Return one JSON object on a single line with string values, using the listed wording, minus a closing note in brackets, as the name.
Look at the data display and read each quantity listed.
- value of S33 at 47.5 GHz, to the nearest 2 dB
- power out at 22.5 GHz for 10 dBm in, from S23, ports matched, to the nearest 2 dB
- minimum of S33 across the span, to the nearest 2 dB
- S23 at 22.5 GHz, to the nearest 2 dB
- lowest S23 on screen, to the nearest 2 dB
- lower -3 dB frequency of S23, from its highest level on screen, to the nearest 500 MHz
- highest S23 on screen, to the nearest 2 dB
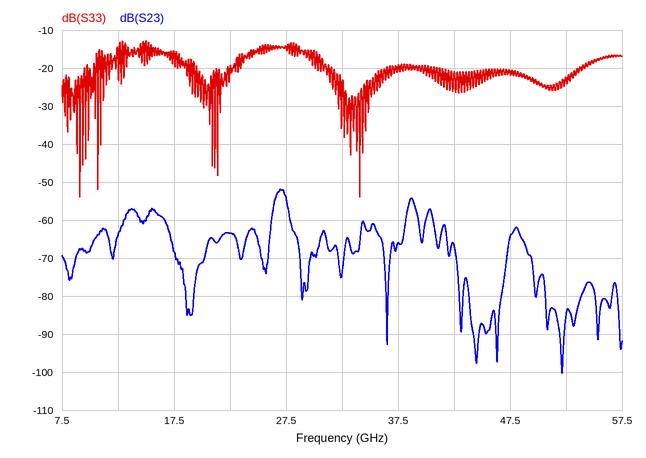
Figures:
{"value of S33 at 47.5 GHz, to the nearest 2 dB": "-22 dB", "power out at 22.5 GHz for 10 dBm in, from S23, ports matched, to the nearest 2 dB": "-54 dBm", "minimum of S33 across the span, to the nearest 2 dB": "-54 dB", "S23 at 22.5 GHz, to the nearest 2 dB": "-64 dB", "lowest S23 on screen, to the nearest 2 dB": "-100 dB", "lower -3 dB frequency of S23, from its highest level on screen, to the nearest 500 MHz": "26.5 GHz", "highest S23 on screen, to the nearest 2 dB": "-52 dB"}
